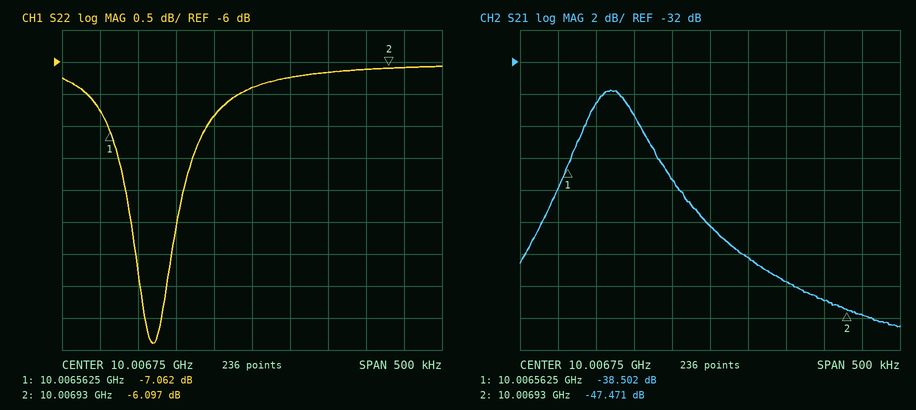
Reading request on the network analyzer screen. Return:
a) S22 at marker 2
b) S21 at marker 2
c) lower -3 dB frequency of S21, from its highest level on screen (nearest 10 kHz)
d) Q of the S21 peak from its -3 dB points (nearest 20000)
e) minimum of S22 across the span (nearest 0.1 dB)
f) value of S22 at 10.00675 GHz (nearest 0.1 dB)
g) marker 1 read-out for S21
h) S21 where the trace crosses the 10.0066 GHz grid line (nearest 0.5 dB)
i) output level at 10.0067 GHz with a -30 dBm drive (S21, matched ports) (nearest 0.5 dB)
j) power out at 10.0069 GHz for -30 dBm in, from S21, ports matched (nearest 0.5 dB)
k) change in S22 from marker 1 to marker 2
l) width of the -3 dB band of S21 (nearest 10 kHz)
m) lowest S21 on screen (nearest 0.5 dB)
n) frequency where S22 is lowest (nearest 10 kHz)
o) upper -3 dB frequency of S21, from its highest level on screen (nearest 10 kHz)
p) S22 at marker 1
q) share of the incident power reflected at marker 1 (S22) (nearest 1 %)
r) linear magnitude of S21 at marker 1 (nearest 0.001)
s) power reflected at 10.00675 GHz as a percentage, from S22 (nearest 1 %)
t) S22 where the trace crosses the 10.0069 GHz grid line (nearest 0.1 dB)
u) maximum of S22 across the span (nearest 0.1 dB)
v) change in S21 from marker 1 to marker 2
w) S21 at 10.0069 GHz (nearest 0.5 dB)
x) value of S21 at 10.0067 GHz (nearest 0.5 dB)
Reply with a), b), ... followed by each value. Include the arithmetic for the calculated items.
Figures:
a) -6.097 dB
b) -47.471 dB
c) 10.00658 GHz
d) 10.0066 GHz / 90 kHz ≈ 111185, so 120000 to the nearest 20000
e) -10.4 dB
f) -6.4 dB
g) -38.502 dB
h) -34.5 dB
i) -30 dBm + (-39.5 dB) = -69.5 dBm
j) -30 dBm + (-47.0 dB) = -77.0 dBm
k) -6.097 − (-7.062) = 0.965 dB
l) 10.00667 GHz − 10.00658 GHz = 90 kHz
m) -48.5 dB
n) 10.00662 GHz
o) 10.00667 GHz
p) -7.062 dB
q) 10^(-7.062/10) ≈ 20 %
r) 10^(-38.502/20) ≈ 0.012
s) 10^(-6.4/10) ≈ 23 %
t) -6.1 dB
u) -6.1 dB
v) -47.471 − (-38.502) = -8.969 dB
w) -47.0 dB
x) -39.5 dB
